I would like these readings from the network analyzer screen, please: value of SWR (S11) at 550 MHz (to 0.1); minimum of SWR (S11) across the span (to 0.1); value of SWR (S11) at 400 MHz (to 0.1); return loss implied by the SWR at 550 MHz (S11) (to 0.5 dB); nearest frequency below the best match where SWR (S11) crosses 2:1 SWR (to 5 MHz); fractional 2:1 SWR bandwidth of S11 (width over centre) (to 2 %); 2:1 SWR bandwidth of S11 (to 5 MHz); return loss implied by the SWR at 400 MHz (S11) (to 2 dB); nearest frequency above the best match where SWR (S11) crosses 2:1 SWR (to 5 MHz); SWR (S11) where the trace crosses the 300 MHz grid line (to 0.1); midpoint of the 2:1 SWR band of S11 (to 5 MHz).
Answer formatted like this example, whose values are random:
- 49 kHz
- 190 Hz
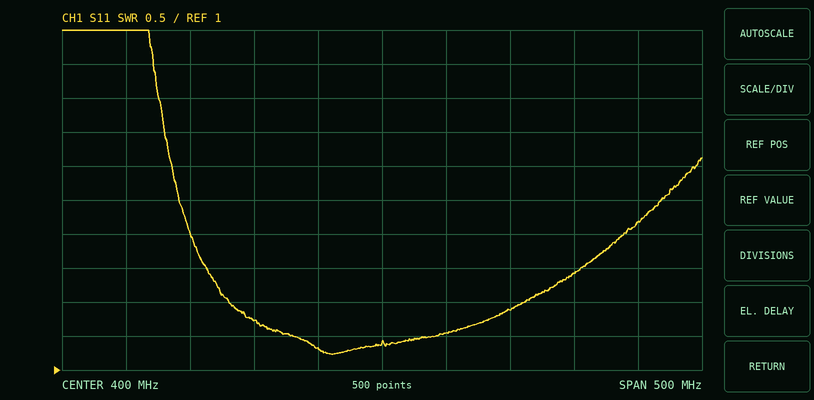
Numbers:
- 2.4
- 1.2
- 1.4
- 7.5 dB
- 280 MHz
- 58 %
- 230 MHz
- 16 dB
- 510 MHz
- 1.7
- 395 MHz
